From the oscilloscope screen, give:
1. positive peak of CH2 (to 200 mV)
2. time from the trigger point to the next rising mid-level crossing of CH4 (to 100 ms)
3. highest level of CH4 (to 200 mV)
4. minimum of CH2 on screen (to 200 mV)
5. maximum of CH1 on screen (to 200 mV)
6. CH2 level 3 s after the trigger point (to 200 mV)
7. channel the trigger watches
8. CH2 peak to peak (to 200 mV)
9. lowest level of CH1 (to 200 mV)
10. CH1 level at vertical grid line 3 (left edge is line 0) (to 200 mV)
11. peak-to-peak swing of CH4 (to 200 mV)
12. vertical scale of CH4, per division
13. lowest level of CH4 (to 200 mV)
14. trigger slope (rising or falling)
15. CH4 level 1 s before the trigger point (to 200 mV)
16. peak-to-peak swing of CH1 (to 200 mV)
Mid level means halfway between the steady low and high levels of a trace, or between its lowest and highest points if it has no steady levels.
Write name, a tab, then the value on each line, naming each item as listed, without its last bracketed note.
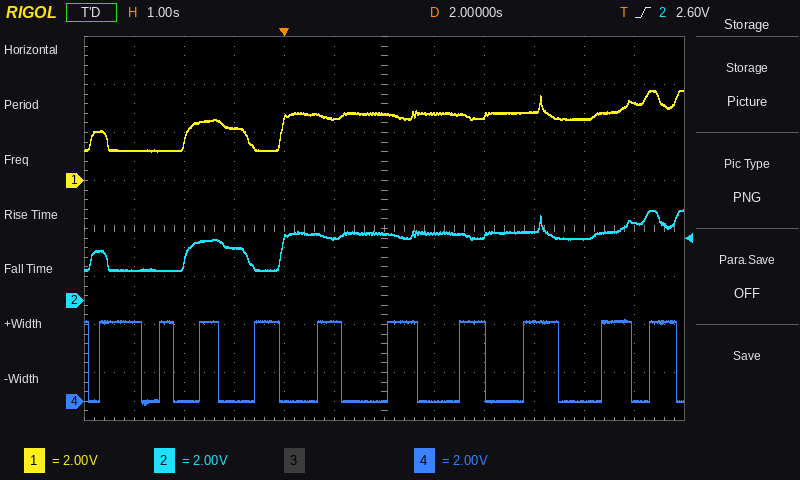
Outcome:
positive peak of CH2	3.8 V
time from the trigger point to the next rising mid-level crossing of CH4	700 ms
highest level of CH4	3.4 V
minimum of CH2 on screen	1.2 V
maximum of CH1 on screen	3.8 V
CH2 level 3 s after the trigger point	2.8 V
channel the trigger watches	CH2
CH2 peak to peak	2.6 V
lowest level of CH1	1.2 V
CH1 level at vertical grid line 3 (left edge is line 0)	2.2 V
peak-to-peak swing of CH4	3.6 V
vertical scale of CH4, per division	2 V
lowest level of CH4	-200 mV
trigger slope	rising
CH4 level 1 s before the trigger point	0.0 V
peak-to-peak swing of CH1	2.6 V
